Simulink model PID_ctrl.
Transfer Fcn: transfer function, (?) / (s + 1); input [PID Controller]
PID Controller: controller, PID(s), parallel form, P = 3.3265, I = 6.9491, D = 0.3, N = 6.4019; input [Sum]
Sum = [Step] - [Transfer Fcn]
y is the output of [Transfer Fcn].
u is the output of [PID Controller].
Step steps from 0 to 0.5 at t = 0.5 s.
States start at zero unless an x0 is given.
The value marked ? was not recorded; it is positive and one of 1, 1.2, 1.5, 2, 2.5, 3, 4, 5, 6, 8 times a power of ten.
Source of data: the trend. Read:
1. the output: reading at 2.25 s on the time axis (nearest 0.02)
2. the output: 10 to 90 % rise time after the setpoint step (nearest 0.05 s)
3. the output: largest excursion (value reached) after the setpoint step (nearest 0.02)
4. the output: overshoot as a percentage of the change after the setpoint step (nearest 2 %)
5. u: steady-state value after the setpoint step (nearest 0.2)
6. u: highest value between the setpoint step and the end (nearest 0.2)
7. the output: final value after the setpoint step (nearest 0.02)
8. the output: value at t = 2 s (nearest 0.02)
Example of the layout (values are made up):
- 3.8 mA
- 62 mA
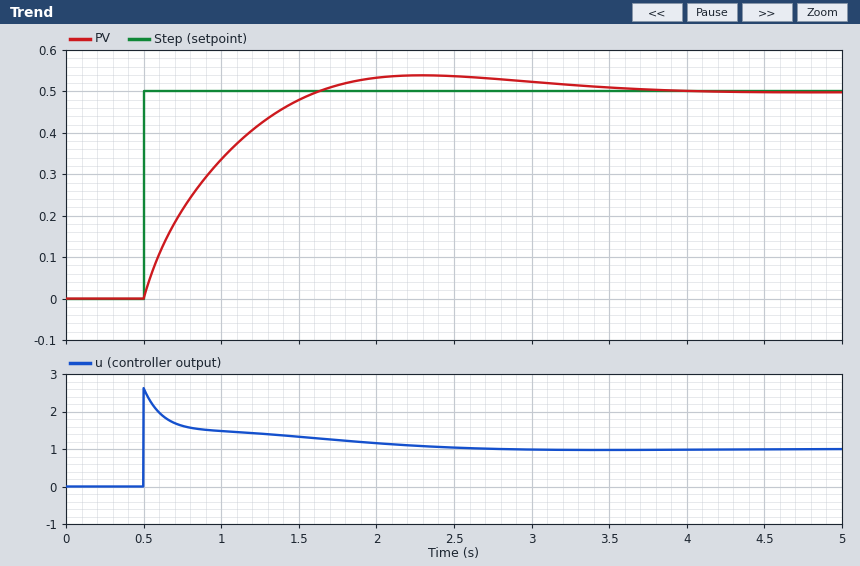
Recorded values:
- 0.54
- 0.80 s
- 0.54
- 8 %
- 1.0
- 2.6
- 0.50
- 0.54
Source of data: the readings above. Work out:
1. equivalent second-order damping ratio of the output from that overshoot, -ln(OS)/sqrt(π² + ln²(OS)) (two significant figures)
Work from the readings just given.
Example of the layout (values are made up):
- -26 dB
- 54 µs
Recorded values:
- 0.63
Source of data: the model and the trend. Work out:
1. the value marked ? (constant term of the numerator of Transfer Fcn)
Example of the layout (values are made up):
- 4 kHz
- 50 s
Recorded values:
- 0.5
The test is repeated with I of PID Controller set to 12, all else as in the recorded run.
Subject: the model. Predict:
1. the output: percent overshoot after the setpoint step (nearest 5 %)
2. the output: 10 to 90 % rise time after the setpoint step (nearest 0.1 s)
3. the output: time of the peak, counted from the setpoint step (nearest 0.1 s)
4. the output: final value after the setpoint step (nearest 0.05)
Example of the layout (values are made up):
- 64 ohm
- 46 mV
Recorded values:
- 15 %
- 0.6 s
- 1.3 s
- 0.50
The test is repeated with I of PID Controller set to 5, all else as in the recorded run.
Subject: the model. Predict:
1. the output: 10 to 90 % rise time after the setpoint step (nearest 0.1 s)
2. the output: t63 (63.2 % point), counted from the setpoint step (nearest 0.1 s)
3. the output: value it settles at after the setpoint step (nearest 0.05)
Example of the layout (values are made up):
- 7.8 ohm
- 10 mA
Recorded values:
- 1.0 s
- 0.5 s
- 0.50
